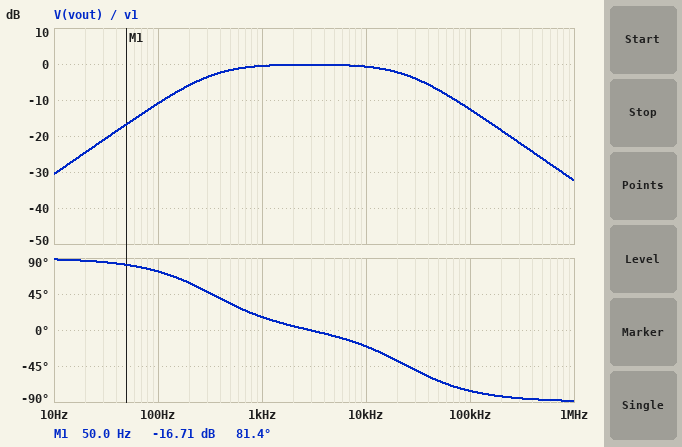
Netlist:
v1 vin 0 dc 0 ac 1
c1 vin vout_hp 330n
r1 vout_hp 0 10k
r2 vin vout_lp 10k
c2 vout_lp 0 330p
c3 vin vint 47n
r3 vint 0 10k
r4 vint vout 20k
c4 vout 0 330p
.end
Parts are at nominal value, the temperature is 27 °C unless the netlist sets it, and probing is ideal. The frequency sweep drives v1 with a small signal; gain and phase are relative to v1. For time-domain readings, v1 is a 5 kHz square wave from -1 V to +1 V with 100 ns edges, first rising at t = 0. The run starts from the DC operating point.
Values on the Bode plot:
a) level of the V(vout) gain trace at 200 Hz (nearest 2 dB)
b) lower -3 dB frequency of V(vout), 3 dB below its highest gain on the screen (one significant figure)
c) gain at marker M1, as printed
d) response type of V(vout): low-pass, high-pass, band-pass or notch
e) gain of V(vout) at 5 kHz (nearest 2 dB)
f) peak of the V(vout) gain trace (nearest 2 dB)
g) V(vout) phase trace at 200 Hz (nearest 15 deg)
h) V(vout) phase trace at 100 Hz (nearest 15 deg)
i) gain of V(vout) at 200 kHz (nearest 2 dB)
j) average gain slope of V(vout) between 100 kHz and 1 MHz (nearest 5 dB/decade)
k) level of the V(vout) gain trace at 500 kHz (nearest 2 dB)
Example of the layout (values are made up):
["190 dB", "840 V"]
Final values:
["-6 dB", "300 Hz", "-16.71 dB", "band-pass", "0 dB", "0 dB", "60 deg", "75 deg", "-18 dB", "-20 dB/decade", "-26 dB"]
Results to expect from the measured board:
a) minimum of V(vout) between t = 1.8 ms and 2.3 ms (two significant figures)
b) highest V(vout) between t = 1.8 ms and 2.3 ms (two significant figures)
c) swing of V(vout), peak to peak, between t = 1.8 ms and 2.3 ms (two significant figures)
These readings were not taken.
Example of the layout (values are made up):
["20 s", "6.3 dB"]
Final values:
["-1.0 V", "1.0 V", "2.1 V"]
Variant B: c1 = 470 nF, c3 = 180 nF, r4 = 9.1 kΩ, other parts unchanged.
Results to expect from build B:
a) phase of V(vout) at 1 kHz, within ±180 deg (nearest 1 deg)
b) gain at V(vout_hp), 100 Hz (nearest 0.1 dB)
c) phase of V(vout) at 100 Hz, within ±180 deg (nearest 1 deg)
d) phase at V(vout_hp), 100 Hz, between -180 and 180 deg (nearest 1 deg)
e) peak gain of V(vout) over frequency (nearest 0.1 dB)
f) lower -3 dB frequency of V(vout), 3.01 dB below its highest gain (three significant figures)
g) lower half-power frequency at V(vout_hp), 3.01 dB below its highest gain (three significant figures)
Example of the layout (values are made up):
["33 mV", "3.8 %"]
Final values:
["4 deg", "-0.5 dB", "41 deg", "19 deg", "0 dB", "88.0 Hz", "33.9 Hz"]
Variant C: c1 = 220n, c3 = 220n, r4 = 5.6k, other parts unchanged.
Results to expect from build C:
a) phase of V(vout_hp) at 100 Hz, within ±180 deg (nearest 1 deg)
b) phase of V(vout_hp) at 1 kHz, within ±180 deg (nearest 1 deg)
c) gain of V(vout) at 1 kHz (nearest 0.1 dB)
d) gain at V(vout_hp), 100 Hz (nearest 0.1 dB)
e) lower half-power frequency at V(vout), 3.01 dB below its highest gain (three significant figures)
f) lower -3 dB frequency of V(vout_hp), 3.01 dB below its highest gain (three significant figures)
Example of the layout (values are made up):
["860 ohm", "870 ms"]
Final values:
["36 deg", "4 deg", "0 dB", "-1.8 dB", "72.1 Hz", "72.3 Hz"]
